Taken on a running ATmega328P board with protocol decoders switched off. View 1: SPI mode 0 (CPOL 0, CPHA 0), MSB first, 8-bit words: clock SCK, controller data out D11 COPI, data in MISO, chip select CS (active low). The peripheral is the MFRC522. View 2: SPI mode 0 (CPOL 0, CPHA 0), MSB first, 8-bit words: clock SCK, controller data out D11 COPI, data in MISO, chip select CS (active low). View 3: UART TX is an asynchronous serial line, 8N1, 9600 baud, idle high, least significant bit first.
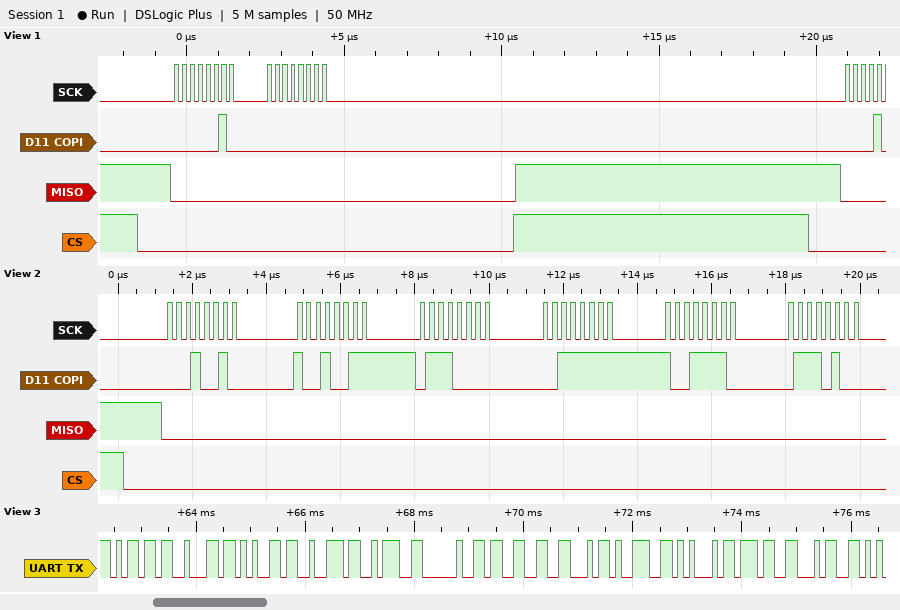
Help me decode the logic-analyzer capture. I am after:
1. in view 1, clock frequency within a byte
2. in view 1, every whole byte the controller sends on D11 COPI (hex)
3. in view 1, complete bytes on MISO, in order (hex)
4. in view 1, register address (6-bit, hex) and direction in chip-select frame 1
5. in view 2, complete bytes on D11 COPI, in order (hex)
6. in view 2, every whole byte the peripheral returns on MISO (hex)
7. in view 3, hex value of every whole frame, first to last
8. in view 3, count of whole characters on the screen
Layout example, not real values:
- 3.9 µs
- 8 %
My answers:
- 4 MHz
- 0x02 0x00
- 0x00 0x00
- 0x01 write
- 0x12 0x93 0x70 0x3F 0x9E 0x74
- 0x00 0x00 0x00 0x00 0x00 0x00
- 6D 62 65 72 3A 20 33 46 39 45 37 34
- 12
